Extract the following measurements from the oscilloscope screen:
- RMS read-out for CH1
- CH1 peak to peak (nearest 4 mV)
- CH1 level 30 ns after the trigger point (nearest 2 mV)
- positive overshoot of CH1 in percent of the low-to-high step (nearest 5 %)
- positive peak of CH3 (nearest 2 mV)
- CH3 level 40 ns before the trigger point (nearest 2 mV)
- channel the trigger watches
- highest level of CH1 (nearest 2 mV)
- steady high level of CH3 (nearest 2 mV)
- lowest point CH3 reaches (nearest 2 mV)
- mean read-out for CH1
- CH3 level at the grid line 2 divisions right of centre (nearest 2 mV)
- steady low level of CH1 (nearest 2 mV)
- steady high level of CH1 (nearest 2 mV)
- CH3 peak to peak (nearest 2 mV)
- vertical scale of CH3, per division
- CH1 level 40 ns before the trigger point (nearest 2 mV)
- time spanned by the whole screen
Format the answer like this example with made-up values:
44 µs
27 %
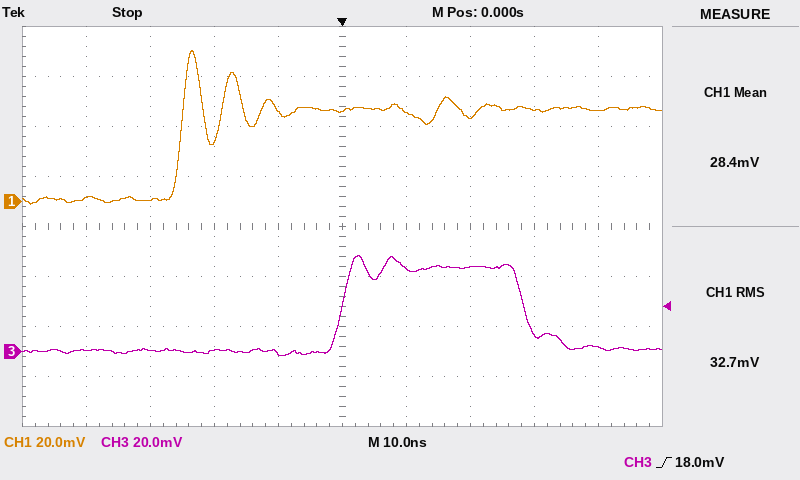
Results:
32.7 mV
60 mV
36 mV
65 %
38 mV
0 mV
CH3
60 mV
34 mV
-2 mV
28.4 mV
34 mV
0 mV
38 mV
40 mV
20 mV
2 mV
100 ns
